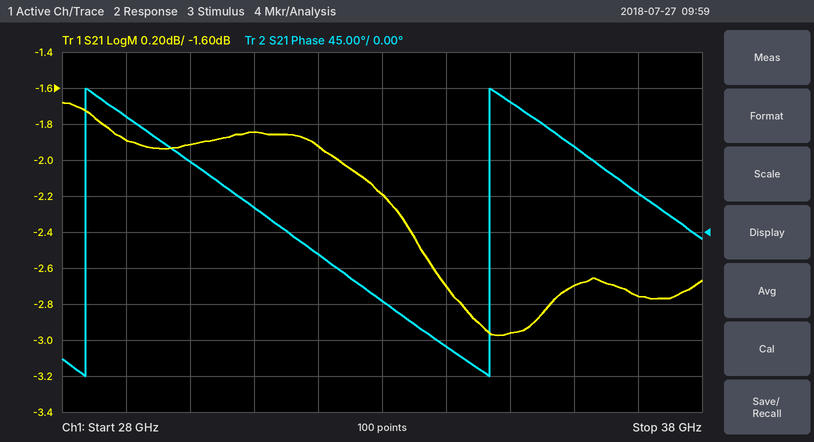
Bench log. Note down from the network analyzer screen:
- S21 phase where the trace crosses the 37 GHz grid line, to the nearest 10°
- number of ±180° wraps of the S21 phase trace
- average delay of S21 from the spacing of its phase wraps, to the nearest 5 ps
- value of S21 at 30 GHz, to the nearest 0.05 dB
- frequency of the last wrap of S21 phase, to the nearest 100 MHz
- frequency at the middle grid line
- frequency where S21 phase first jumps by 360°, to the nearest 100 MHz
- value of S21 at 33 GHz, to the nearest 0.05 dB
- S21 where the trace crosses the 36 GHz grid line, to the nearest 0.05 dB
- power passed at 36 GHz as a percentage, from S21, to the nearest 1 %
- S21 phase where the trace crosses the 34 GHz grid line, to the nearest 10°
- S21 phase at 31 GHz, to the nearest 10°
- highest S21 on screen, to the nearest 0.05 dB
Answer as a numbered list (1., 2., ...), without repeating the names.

1. 50°
2. 2
3. 160 ps
4. -1.90 dB
5. 34.7 GHz
6. 33 GHz
7. 28.4 GHz
8. -2.20 dB
9. -2.70 dB
10. 54 %
11. -140°
12. 30°
13. -1.70 dB
